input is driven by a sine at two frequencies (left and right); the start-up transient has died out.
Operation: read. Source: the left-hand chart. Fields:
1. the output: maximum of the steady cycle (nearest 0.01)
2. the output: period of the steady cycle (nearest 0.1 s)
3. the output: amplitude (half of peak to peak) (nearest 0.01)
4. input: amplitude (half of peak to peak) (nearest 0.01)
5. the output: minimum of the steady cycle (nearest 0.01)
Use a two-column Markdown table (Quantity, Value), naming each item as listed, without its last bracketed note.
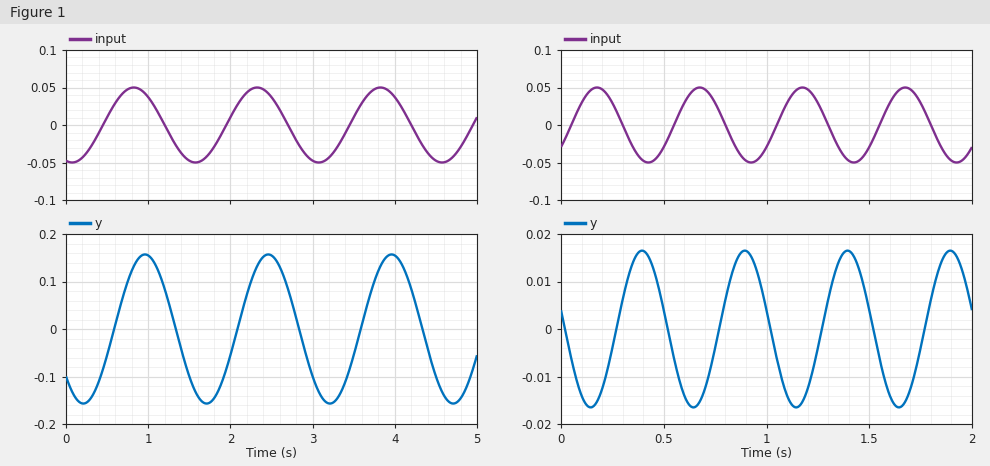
| Quantity | Value |
|---|---|
| the output: maximum of the steady cycle | 0.16 |
| the output: period of the steady cycle | 1.5 s |
| the output: amplitude (half of peak to peak) | 0.16 |
| input: amplitude (half of peak to peak) | 0.05 |
| the output: minimum of the steady cycle | -0.16 |
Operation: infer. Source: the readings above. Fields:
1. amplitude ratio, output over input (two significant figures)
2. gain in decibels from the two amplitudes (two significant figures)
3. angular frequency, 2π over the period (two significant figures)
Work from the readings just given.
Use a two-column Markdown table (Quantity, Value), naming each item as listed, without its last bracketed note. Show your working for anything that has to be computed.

| Quantity | Value |
|---|---|
| amplitude ratio, output over input | 0.16 / 0.05 = 3.2 |
| gain in decibels from the two amplitudes | 20 log10(0.16 / 0.05) = 10 dB |
| angular frequency, 2π over the period | 2π / 1.5 = 4.2 rad/s |
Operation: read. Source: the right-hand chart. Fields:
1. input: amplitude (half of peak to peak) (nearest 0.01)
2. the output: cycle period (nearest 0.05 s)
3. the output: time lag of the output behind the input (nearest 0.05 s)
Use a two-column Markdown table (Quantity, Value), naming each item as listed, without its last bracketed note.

| Quantity | Value |
|---|---|
| input: amplitude (half of peak to peak) | 0.05 |
| the output: cycle period | 0.50 s |
| the output: time lag of the output behind the input | 0.20 s |
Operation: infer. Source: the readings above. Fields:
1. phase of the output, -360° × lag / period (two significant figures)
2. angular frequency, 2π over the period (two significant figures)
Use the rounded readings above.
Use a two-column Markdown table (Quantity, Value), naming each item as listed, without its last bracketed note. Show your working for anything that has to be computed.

| Quantity | Value |
|---|---|
| phase of the output, -360° × lag / period | -360 × 0.2 / 0.5 = -140° |
| angular frequency, 2π over the period | 2π / 0.5 = 13 rad/s |
